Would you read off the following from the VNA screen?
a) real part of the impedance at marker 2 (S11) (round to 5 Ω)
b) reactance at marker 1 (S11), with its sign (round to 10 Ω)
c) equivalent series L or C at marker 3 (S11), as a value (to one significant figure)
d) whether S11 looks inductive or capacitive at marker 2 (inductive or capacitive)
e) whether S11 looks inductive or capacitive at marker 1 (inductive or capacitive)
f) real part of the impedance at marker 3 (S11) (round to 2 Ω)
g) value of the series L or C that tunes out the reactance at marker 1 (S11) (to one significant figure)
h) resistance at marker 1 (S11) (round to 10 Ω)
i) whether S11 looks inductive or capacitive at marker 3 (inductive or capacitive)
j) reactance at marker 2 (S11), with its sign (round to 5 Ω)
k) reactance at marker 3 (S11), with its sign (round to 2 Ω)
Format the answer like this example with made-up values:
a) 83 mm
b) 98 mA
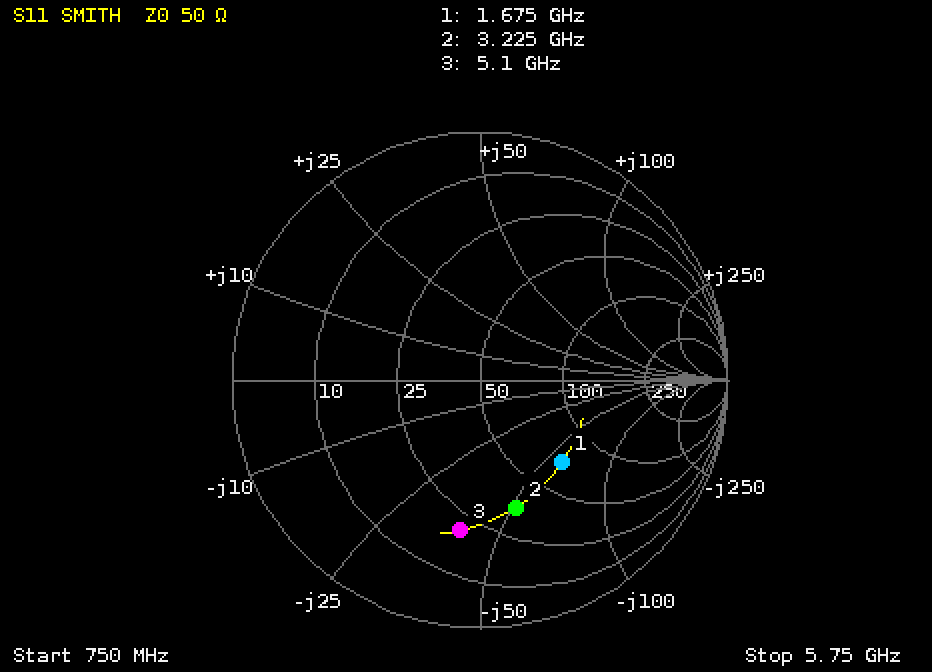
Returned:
a) 35 Ω
b) -60 Ω
c) 800 fF
d) capacitive
e) capacitive
f) 20 Ω
g) 6 nH
h) 70 Ω
i) capacitive
j) -50 Ω
k) -40 Ω
